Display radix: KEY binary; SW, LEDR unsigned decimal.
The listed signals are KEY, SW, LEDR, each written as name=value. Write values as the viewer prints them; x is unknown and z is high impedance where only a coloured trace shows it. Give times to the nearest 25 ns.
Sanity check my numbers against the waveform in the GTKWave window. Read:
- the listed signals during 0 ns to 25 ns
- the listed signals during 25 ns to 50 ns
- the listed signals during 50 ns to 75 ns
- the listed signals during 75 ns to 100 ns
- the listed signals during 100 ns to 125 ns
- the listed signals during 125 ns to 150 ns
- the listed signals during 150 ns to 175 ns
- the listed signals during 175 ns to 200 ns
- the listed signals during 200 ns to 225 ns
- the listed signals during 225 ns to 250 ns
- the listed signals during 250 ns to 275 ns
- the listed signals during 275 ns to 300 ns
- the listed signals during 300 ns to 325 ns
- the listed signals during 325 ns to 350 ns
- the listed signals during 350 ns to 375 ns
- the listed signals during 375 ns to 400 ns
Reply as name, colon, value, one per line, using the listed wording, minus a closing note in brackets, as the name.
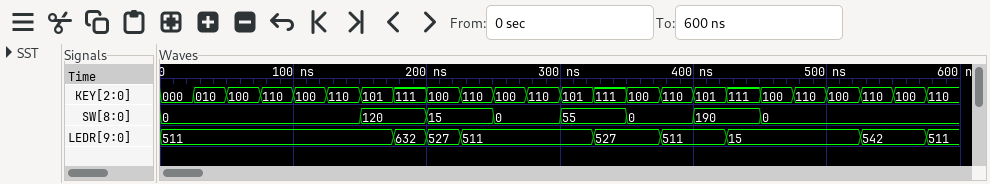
the listed signals during 0 ns to 25 ns: KEY=000, SW=0, LEDR=511
the listed signals during 25 ns to 50 ns: KEY=010, SW=0, LEDR=511
the listed signals during 50 ns to 75 ns: KEY=100, SW=0, LEDR=511
the listed signals during 75 ns to 100 ns: KEY=110, SW=0, LEDR=511
the listed signals during 100 ns to 125 ns: KEY=100, SW=0, LEDR=511
the listed signals during 125 ns to 150 ns: KEY=110, SW=0, LEDR=511
the listed signals during 150 ns to 175 ns: KEY=101, SW=120, LEDR=511
the listed signals during 175 ns to 200 ns: KEY=111, SW=120, LEDR=632
the listed signals during 200 ns to 225 ns: KEY=100, SW=15, LEDR=527
the listed signals during 225 ns to 250 ns: KEY=110, SW=15, LEDR=511
the listed signals during 250 ns to 275 ns: KEY=100, SW=0, LEDR=511
the listed signals during 275 ns to 300 ns: KEY=110, SW=0, LEDR=511
the listed signals during 300 ns to 325 ns: KEY=101, SW=55, LEDR=511
the listed signals during 325 ns to 350 ns: KEY=111, SW=55, LEDR=527
the listed signals during 350 ns to 375 ns: KEY=100, SW=0, LEDR=527
the listed signals during 375 ns to 400 ns: KEY=110, SW=0, LEDR=511
